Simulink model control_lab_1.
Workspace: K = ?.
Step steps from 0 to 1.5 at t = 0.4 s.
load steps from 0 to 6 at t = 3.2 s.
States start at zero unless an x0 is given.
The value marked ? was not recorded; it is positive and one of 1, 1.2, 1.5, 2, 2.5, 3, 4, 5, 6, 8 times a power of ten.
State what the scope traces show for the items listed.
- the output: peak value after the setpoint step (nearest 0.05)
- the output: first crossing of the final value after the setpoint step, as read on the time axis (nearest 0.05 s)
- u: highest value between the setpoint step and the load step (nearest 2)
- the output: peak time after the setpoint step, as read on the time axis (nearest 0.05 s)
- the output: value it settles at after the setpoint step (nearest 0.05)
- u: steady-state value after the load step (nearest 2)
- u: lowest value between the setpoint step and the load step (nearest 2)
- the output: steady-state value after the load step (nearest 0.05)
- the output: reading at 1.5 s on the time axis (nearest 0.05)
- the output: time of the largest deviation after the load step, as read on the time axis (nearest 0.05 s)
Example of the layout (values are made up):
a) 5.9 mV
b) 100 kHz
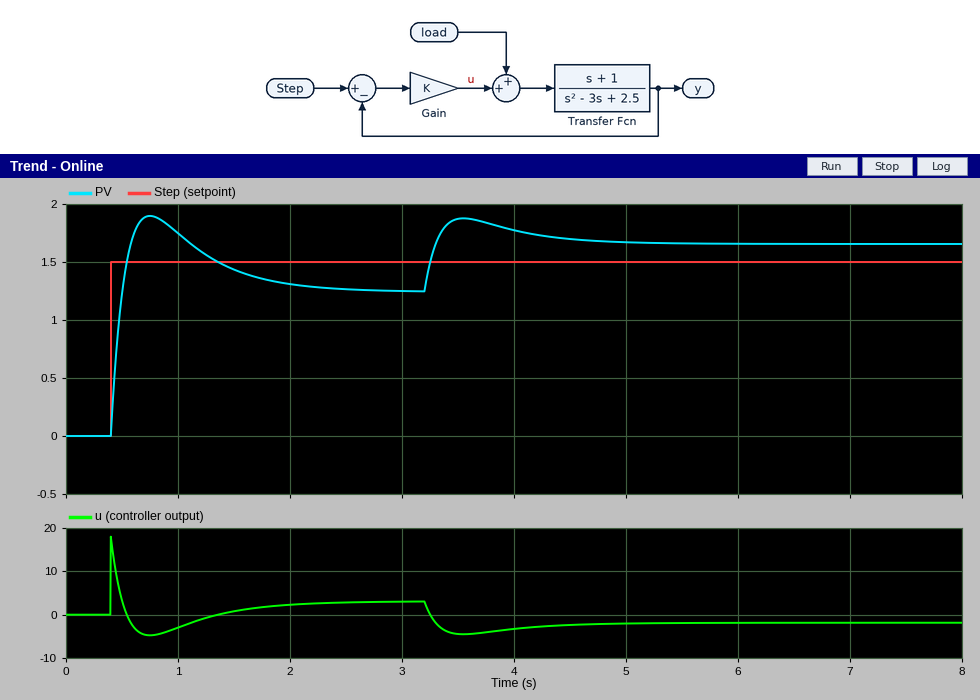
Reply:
a) 1.90
b) 0.50 s
c) 18
d) 0.75 s
e) 1.25
f) -2
g) -4
h) 1.65
i) 1.45
j) 3.55 s
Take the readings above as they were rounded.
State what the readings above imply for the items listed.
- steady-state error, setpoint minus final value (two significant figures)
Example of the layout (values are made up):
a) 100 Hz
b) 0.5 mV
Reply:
a) 0.25
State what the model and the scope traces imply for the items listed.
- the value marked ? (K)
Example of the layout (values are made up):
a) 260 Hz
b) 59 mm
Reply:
a) 12
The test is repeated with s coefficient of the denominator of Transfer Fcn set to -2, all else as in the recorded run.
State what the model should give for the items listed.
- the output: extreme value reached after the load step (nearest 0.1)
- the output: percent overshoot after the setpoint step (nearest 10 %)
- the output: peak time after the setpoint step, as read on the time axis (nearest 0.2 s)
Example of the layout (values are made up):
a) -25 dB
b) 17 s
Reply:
a) 1.8
b) 40 %
c) 0.8 s
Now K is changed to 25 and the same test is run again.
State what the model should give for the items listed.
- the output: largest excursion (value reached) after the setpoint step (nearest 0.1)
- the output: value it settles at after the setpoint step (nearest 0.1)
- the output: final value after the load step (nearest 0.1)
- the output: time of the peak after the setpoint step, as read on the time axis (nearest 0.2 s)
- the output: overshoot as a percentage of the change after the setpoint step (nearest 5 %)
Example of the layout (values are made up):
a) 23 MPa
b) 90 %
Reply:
a) 1.7
b) 1.4
c) 1.6
d) 0.6 s
e) 25 %
